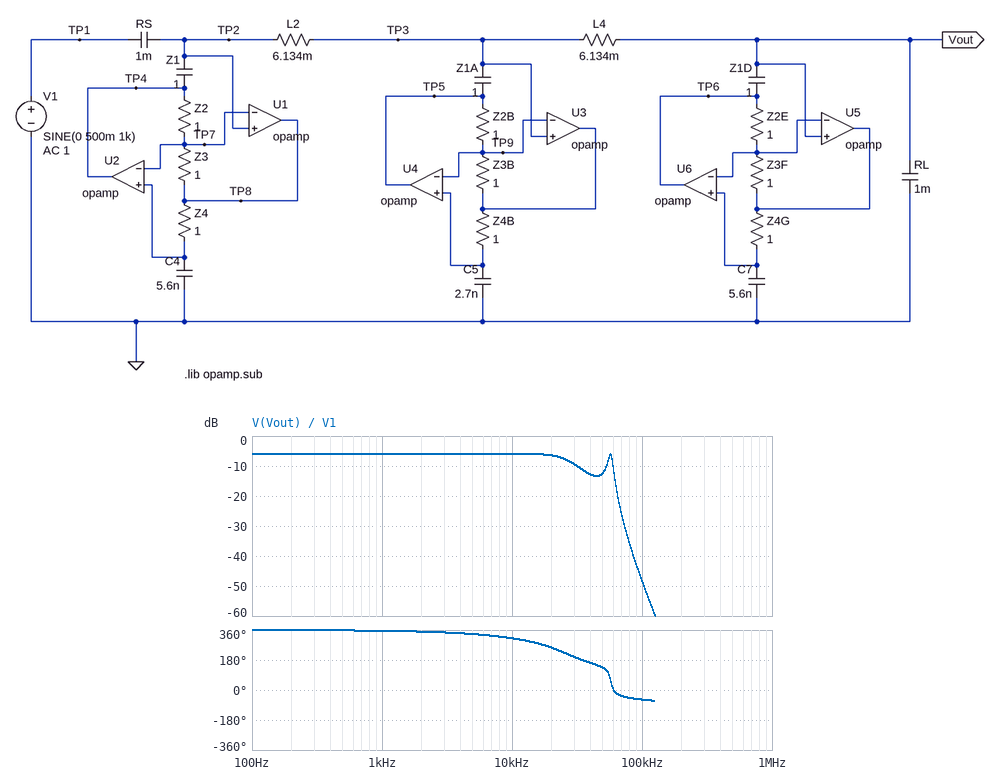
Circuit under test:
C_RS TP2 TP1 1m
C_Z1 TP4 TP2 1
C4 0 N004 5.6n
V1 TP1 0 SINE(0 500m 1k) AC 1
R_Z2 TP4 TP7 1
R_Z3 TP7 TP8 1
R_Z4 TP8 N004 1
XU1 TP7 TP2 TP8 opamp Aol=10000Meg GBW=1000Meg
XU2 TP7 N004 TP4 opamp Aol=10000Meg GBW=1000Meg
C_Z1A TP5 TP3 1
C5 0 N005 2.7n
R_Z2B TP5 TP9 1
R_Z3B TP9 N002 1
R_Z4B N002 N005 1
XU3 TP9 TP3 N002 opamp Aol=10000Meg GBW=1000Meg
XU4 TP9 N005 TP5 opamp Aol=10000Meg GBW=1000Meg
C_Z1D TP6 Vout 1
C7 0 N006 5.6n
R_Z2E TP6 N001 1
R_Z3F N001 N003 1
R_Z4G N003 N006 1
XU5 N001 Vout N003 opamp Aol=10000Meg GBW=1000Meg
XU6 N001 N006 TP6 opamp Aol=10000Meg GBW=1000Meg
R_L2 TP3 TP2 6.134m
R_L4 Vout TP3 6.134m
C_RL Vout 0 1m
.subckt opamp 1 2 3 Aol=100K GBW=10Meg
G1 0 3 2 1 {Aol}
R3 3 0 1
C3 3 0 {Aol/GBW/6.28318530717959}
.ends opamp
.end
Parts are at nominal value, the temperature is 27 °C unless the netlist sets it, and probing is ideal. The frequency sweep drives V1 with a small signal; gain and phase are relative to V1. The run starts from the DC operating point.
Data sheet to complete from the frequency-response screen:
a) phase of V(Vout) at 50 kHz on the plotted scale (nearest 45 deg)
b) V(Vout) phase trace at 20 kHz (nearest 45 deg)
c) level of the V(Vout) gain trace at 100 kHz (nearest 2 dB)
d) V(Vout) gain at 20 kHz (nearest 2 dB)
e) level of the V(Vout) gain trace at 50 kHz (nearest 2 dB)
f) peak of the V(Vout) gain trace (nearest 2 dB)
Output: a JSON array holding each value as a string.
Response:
["135 deg", "270 deg", "-48 dB", "-6 dB", "-12 dB", "-6 dB"]
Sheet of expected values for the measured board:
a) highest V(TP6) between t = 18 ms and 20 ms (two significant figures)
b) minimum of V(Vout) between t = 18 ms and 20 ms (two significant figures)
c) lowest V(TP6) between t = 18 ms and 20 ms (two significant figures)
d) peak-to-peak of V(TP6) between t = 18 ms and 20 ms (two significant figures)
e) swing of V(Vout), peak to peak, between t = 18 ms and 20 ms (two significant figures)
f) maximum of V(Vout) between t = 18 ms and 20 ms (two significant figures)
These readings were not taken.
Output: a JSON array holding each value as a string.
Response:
["250 mV", "-250 mV", "-250 mV", "500 mV", "500 mV", "250 mV"]
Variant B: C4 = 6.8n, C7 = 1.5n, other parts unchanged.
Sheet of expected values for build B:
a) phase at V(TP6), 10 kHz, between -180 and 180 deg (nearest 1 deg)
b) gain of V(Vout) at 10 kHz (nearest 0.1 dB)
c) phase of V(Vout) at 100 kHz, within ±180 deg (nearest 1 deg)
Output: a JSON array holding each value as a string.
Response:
["-45 deg", "-6.1 dB", "-26 deg"]
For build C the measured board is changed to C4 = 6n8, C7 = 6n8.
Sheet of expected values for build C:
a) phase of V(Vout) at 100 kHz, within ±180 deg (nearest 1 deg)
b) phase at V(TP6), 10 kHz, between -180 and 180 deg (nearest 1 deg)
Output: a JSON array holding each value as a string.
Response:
["-63 deg", "-54 deg"]
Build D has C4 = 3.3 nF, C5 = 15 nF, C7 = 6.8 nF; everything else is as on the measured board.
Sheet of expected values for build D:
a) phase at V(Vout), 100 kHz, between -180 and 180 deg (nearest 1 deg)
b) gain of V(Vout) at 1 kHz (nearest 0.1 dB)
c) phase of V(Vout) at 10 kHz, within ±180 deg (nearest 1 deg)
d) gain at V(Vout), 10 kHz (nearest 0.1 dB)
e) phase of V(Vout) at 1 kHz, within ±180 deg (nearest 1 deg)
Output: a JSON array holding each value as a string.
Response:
["-50 deg", "-6.0 dB", "-67 deg", "-6.5 dB", "-7 deg"]
